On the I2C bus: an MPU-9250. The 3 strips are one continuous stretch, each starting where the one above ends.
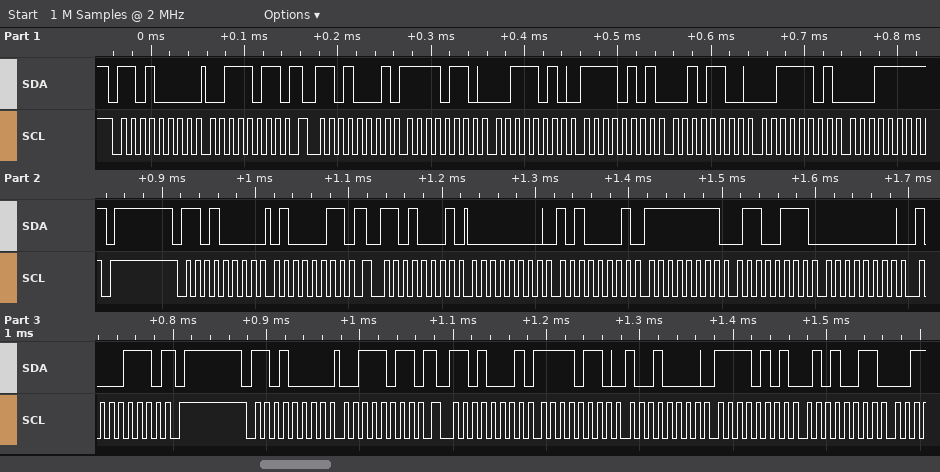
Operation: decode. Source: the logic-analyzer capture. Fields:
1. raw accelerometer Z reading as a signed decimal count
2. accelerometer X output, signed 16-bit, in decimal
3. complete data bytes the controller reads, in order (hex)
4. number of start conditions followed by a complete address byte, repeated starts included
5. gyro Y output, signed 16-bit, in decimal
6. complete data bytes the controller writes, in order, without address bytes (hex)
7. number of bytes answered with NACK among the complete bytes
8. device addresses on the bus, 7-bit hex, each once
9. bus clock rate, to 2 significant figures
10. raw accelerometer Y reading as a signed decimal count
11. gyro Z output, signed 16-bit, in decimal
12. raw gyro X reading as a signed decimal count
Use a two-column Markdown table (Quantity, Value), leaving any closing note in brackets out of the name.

| Quantity | Value |
|---|---|
| raw accelerometer Z reading as a signed decimal count | 15647 |
| accelerometer X output, signed 16-bit, in decimal | -2502 |
| complete data bytes the controller reads, in order | F6 3A F5 2C 3D 1F 00 A1 FF 67 00 8E F6 90 F5 53 |
| number of start conditions followed by a complete address byte, repeated starts included | 6 |
| gyro Y output, signed 16-bit, in decimal | -153 |
| complete data bytes the controller writes, in order, without address bytes | 3B 43 3B |
| number of bytes answered with NACK among the complete bytes | 2 |
| device addresses on the bus, 7-bit hex, each once | 0x68 |
| bus clock rate, to 2 significant figures | 100 kHz |
| raw accelerometer Y reading as a signed decimal count | -2772 |
| gyro Z output, signed 16-bit, in decimal | 142 |
| raw gyro X reading as a signed decimal count | 161 |
